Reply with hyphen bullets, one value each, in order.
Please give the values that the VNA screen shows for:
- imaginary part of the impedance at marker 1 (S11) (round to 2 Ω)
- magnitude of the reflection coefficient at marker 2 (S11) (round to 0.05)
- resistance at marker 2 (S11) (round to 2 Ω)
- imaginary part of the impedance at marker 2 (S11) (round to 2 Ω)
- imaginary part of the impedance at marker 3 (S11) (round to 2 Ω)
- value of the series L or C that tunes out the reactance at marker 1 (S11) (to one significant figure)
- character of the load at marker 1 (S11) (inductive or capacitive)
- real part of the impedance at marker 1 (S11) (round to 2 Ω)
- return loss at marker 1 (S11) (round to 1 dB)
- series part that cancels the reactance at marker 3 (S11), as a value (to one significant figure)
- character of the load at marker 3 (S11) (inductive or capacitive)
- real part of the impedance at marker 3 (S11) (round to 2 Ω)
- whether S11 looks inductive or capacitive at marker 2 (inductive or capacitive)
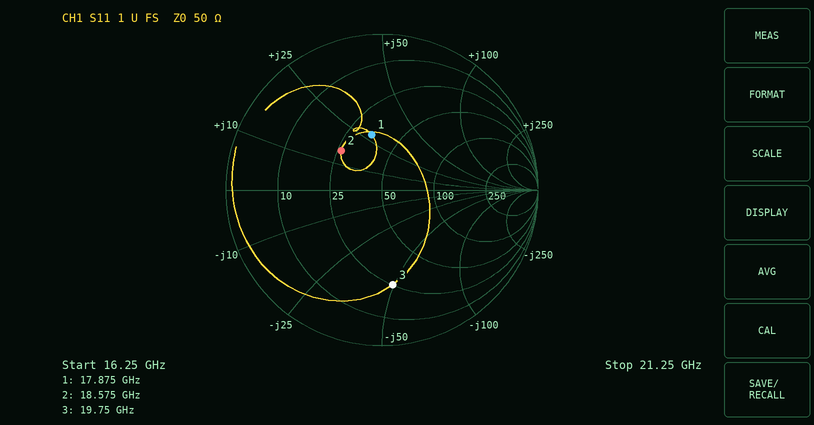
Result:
- +28 Ω
- 0.35
- 26 Ω
- +16 Ω
- -50 Ω
- 300 fF
- inductive
- 34 Ω
- 9 dB
- 400 pH
- capacitive
- 26 Ω
- inductive
